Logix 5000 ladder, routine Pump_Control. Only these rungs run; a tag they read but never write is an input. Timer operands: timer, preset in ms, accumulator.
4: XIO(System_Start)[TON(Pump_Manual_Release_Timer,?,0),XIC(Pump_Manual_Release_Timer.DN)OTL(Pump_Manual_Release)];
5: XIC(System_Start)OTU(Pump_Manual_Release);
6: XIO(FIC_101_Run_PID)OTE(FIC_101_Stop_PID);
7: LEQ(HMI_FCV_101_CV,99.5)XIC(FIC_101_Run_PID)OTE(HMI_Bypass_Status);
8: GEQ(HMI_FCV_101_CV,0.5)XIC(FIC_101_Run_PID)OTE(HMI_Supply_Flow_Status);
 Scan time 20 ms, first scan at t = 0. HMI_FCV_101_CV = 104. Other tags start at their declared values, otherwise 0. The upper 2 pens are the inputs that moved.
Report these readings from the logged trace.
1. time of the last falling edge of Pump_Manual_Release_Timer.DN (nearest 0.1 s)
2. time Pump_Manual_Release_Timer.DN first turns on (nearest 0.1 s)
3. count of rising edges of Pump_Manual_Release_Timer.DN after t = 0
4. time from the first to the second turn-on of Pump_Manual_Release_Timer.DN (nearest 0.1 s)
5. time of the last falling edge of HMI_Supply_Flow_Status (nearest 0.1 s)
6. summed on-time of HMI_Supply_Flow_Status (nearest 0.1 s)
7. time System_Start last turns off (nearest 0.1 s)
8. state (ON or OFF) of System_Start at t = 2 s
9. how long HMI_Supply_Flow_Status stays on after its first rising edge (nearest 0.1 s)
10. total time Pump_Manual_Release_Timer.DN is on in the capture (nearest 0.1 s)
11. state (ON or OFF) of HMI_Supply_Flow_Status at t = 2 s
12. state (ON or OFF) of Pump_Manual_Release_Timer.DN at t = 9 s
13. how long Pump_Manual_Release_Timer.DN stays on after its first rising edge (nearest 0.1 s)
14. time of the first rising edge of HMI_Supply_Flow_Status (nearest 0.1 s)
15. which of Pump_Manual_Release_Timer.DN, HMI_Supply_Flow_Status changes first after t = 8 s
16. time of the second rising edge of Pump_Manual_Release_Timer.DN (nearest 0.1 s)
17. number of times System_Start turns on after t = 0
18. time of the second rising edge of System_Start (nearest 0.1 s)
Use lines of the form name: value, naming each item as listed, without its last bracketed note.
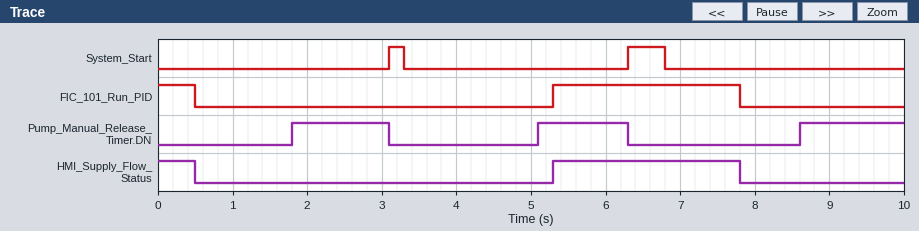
time of the last falling edge of Pump_Manual_Release_Timer.DN: 6.3 s
time Pump_Manual_Release_Timer.DN first turns on: 1.8 s
count of rising edges of Pump_Manual_Release_Timer.DN after t = 0: 3
time from the first to the second turn-on of Pump_Manual_Release_Timer.DN: 3.3 s
time of the last falling edge of HMI_Supply_Flow_Status: 7.8 s
summed on-time of HMI_Supply_Flow_Status: 3.0 s
time System_Start last turns off: 6.8 s
state (ON or OFF) of System_Start at t = 2 s: OFF
how long HMI_Supply_Flow_Status stays on after its first rising edge: 2.5 s
total time Pump_Manual_Release_Timer.DN is on in the capture: 3.9 s
state (ON or OFF) of HMI_Supply_Flow_Status at t = 2 s: OFF
state (ON or OFF) of Pump_Manual_Release_Timer.DN at t = 9 s: ON
how long Pump_Manual_Release_Timer.DN stays on after its first rising edge: 1.3 s
time of the first rising edge of HMI_Supply_Flow_Status: 5.3 s
which of Pump_Manual_Release_Timer.DN, HMI_Supply_Flow_Status changes first after t = 8 s: Pump_Manual_Release_Timer.DN
time of the second rising edge of Pump_Manual_Release_Timer.DN: 5.1 s
number of times System_Start turns on after t = 0: 2
time of the second rising edge of System_Start: 6.3 s
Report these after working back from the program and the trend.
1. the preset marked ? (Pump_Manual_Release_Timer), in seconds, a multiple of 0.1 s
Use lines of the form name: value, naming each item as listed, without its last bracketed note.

the preset marked ? (Pump_Manual_Release_Timer), in seconds, a multiple of 0.1 s: 1.8 s
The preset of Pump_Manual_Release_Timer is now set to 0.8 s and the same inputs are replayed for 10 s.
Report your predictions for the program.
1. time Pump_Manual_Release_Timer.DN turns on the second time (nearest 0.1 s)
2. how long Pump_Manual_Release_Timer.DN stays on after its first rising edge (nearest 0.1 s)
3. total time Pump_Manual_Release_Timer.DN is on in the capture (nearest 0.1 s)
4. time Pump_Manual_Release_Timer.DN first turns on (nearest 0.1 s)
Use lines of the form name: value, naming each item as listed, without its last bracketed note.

time Pump_Manual_Release_Timer.DN turns on the second time: 4.1 s
how long Pump_Manual_Release_Timer.DN stays on after its first rising edge: 2.3 s
total time Pump_Manual_Release_Timer.DN is on in the capture: 6.9 s
time Pump_Manual_Release_Timer.DN first turns on: 0.8 s
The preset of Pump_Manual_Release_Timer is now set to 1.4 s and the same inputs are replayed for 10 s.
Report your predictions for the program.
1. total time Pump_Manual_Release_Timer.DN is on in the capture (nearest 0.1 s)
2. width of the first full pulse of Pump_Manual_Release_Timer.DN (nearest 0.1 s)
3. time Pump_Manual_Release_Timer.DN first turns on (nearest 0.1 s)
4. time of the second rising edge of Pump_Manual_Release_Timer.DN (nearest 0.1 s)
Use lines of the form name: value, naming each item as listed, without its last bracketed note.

total time Pump_Manual_Release_Timer.DN is on in the capture: 5.1 s
width of the first full pulse of Pump_Manual_Release_Timer.DN: 1.7 s
time Pump_Manual_Release_Timer.DN first turns on: 1.4 s
time of the second rising edge of Pump_Manual_Release_Timer.DN: 4.7 s
